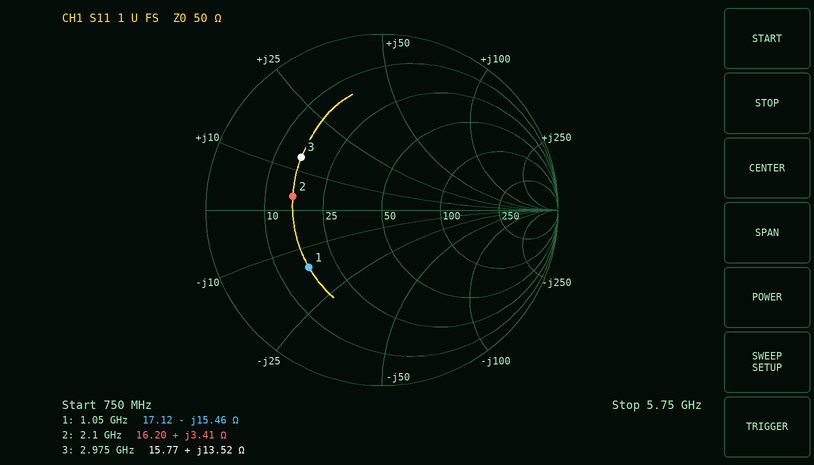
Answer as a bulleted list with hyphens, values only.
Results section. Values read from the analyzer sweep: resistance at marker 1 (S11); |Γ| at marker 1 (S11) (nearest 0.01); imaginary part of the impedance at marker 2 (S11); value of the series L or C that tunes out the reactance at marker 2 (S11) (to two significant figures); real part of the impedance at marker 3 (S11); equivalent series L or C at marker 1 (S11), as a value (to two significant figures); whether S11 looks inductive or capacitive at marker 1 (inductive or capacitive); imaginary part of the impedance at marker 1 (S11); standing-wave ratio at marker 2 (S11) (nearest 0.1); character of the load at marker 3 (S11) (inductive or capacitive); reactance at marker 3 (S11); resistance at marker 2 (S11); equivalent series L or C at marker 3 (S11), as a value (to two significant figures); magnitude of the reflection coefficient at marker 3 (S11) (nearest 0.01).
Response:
- 17.12 Ω
- 0.53
- +3.41 Ω
- 22 pF
- 15.77 Ω
- 9.8 pF
- capacitive
- -15.46 Ω
- 3.1
- inductive
- +13.52 Ω
- 16.20 Ω
- 720 pH
- 0.55
